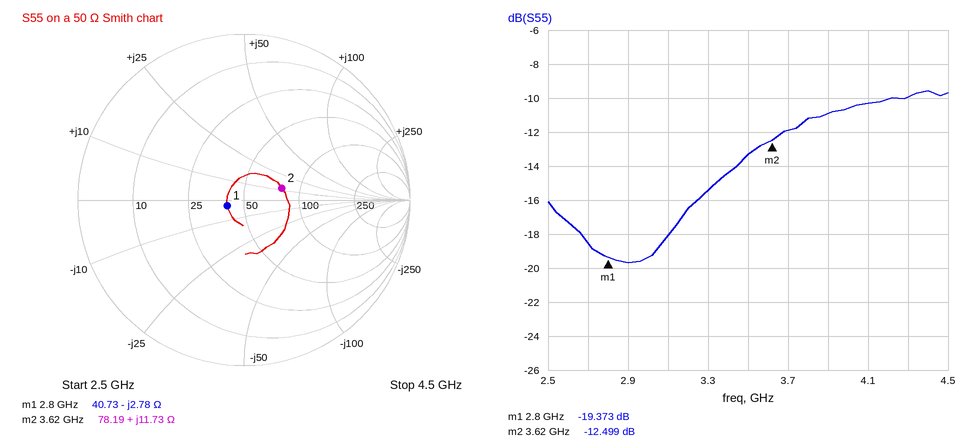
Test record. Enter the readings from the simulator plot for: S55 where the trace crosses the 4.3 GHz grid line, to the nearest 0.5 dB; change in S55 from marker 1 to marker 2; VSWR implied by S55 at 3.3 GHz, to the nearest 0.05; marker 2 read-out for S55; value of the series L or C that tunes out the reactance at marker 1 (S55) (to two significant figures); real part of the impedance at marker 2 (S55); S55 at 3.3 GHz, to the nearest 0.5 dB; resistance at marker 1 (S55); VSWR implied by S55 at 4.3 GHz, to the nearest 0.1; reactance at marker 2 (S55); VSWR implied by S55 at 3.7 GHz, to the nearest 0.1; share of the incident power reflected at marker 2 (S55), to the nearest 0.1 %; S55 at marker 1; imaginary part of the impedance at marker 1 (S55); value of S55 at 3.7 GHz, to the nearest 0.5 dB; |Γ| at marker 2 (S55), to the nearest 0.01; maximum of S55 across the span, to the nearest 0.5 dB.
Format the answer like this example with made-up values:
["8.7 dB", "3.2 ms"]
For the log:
["-10.0 dB", "6.874 dB", "1.40", "-12.499 dB", "160 pH", "78.19 Ω", "-15.5 dB", "40.73 Ω", "1.9", "+11.73 Ω", "1.7", "5.6 %", "-19.373 dB", "-2.78 Ω", "-12.0 dB", "0.24", "-9.5 dB"]
